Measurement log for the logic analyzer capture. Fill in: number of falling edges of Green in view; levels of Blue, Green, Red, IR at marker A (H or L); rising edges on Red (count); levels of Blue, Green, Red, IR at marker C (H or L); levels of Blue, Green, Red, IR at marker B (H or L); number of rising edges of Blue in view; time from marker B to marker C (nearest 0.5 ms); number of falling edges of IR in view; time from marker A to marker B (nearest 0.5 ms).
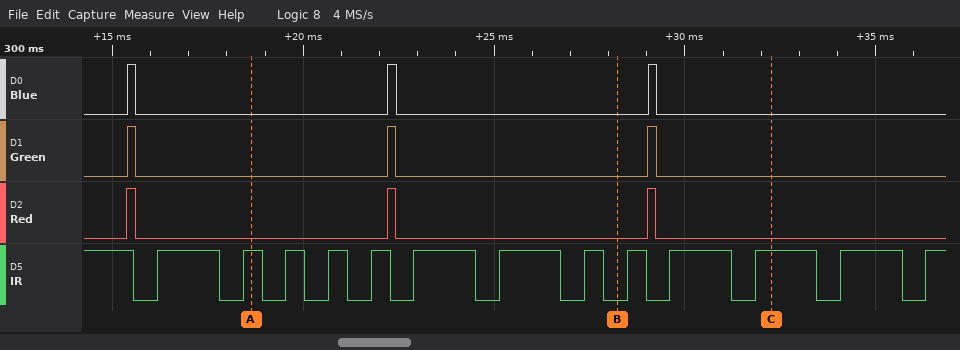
3
Blue=L, Green=L, Red=L, IR=H
3
Blue=L, Green=L, Red=L, IR=H
Blue=L, Green=L, Red=L, IR=L
3
4 ms
13
9.5 ms
